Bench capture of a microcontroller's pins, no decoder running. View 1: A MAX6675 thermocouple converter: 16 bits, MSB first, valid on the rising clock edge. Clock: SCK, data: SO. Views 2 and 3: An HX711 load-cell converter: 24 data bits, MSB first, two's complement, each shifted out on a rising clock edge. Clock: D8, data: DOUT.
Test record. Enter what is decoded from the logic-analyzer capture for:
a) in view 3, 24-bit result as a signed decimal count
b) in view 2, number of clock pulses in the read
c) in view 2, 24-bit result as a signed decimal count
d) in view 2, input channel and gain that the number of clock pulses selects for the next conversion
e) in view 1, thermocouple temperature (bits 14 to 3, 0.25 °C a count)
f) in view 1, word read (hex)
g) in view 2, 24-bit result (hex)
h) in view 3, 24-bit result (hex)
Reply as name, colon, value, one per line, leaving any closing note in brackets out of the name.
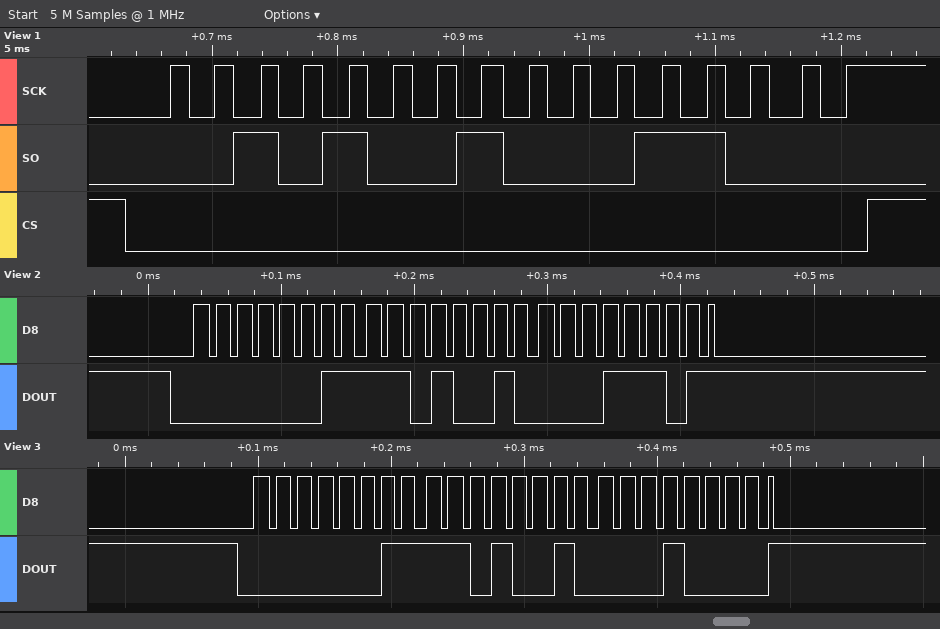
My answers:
in view 3, 24-bit result as a signed decimal count: 250384
in view 2, number of clock pulses in the read: 25
in view 2, 24-bit result as a signed decimal count: 250397
in view 2, input channel and gain that the number of clock pulses selects for the next conversion: channel A, gain 128
in view 1, thermocouple temperature: 328.75 °C
in view 1, word read: 0x2918
in view 2, 24-bit result: 0x03D21D
in view 3, 24-bit result: 0x03D210
